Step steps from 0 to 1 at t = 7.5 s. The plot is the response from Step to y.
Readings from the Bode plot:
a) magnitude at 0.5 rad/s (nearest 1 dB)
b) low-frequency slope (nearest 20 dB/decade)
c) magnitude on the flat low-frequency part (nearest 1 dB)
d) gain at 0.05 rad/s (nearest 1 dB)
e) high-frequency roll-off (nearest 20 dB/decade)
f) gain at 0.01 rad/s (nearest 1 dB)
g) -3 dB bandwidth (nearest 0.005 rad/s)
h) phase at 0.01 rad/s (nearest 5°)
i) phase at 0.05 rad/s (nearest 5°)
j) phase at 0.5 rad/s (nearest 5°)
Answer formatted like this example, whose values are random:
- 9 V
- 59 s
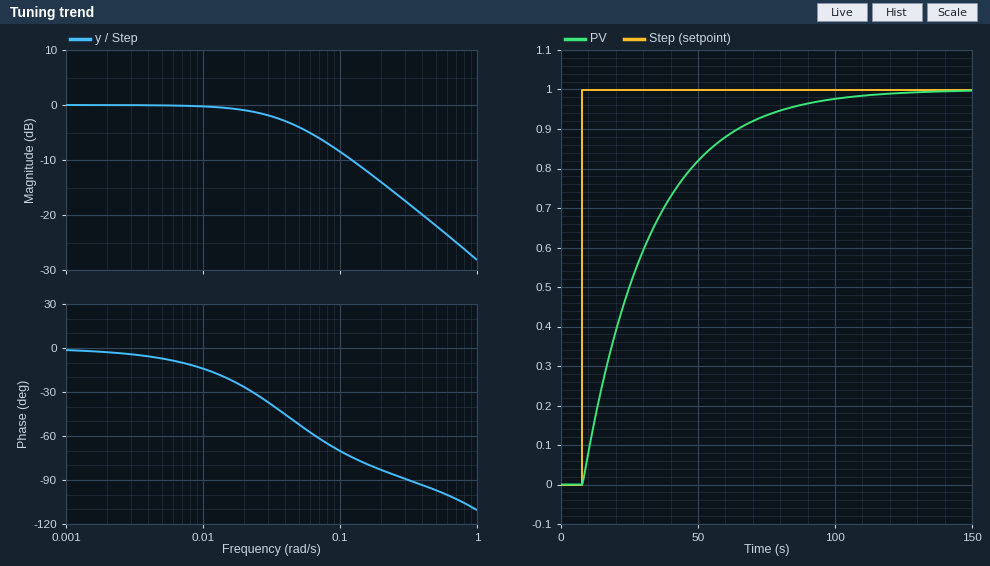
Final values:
- -22 dB
- 0 dB/decade
- 0 dB
- -4 dB
- -20 dB/decade
- 0 dB
- 0.040 rad/s
- -15°
- -50°
- -95°
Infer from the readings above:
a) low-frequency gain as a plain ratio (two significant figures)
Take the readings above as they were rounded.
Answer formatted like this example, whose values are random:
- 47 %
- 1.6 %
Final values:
- 1.0
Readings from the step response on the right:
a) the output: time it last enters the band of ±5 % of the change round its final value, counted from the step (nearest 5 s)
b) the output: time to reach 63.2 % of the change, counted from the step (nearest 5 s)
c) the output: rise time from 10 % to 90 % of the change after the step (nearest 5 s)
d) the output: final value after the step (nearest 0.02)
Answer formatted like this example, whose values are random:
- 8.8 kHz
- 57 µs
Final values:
- 75 s
- 25 s
- 55 s
- 1.00
